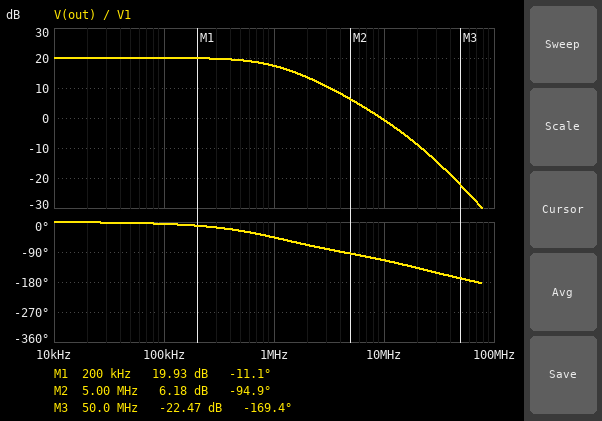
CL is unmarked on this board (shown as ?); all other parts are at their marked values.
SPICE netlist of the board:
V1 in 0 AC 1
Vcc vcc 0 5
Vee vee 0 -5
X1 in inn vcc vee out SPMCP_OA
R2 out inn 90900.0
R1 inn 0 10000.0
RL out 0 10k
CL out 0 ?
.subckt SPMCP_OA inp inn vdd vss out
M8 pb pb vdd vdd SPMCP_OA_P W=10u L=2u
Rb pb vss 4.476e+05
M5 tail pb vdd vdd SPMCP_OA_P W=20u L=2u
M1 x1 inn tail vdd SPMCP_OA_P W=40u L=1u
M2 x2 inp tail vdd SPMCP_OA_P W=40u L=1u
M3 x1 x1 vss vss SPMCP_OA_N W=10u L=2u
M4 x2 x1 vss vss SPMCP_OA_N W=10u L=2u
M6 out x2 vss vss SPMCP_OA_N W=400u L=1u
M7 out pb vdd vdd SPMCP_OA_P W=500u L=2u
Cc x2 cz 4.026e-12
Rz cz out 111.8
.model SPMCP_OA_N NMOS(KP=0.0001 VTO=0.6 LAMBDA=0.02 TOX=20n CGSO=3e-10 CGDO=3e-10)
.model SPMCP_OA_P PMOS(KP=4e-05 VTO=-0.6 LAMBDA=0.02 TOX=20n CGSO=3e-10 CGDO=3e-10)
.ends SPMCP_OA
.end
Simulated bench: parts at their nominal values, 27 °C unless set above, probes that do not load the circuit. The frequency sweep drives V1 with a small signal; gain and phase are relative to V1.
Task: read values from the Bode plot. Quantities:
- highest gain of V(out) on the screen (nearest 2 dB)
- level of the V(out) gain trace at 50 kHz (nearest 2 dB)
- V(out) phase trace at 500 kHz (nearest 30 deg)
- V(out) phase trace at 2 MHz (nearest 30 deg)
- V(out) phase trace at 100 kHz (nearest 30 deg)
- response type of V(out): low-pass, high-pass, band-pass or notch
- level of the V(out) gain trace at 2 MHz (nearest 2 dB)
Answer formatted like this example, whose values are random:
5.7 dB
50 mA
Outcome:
20 dB
20 dB
-30 deg
-60 deg
0 deg
low-pass
14 dB
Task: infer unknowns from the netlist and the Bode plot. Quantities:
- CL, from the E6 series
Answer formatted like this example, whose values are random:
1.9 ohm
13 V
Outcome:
68 pF
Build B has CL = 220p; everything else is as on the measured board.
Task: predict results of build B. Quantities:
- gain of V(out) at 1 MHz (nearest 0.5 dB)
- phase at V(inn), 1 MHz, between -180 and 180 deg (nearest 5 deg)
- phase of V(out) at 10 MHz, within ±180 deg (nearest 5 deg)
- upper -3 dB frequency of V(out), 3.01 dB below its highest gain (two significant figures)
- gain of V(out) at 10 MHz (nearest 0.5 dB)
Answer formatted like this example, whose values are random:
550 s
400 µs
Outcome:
18.0 dB
-50 deg
-150 deg
1.2 MHz
-5.0 dB
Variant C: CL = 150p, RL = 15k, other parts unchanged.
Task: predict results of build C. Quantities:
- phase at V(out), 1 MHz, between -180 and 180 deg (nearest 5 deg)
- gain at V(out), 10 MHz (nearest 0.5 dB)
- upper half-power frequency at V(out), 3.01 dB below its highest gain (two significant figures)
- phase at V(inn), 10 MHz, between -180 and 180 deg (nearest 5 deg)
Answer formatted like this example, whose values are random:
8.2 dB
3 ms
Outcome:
-50 deg
-3.0 dB
1.2 MHz
-155 deg
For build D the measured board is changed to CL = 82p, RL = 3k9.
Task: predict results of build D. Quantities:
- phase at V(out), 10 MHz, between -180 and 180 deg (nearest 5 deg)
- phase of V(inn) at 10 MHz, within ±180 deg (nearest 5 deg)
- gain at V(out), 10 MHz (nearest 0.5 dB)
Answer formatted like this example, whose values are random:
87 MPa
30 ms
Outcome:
-120 deg
-130 deg
-1.0 dB
